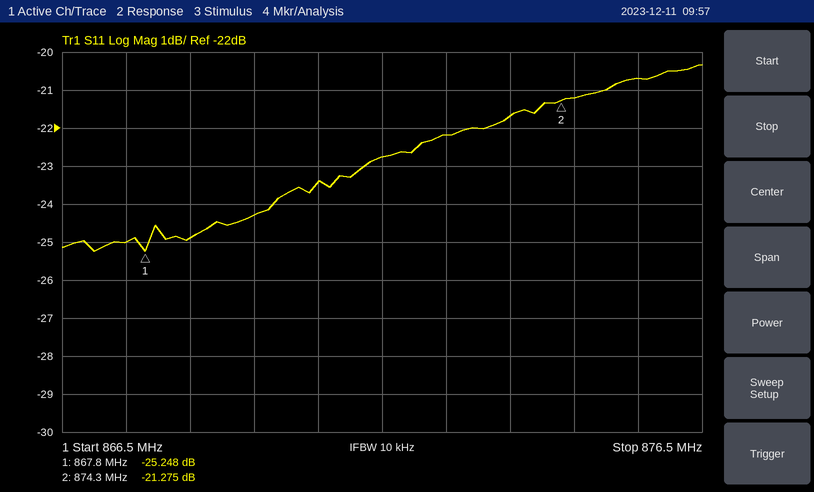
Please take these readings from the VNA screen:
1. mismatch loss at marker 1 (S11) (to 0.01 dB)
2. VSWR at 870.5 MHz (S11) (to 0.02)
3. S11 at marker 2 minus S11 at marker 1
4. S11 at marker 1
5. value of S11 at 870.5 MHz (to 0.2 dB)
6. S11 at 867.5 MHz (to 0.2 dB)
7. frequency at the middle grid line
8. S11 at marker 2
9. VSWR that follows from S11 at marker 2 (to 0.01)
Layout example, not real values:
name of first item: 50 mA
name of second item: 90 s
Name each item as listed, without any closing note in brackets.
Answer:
mismatch loss at marker 1 (S11): 0.01 dB
VSWR at 870.5 MHz (S11): 1.14
S11 at marker 2 minus S11 at marker 1: 3.973 dB
S11 at marker 1: -25.248 dB
value of S11 at 870.5 MHz: -23.4 dB
S11 at 867.5 MHz: -25.0 dB
frequency at the middle grid line: 871.5 MHz
S11 at marker 2: -21.275 dB
VSWR that follows from S11 at marker 2: 1.19
